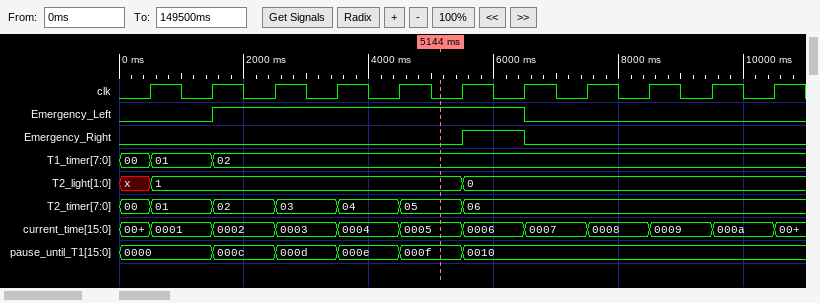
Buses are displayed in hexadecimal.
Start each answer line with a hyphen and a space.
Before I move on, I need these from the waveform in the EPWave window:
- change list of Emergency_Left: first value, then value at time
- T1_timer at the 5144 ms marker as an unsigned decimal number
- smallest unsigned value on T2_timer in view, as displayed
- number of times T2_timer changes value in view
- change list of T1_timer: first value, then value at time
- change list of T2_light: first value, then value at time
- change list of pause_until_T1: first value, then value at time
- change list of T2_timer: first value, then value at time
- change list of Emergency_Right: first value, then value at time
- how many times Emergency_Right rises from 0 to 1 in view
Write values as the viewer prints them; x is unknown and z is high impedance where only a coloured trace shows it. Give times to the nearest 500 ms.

- 0, 1 at 1500 ms, 0 at 6500 ms
- 2
- 00
- 6
- 00, 01 at 500 ms, 02 at 1500 ms
- x, 1 at 500 ms, 0 at 5500 ms
- 0000, 000c at 1500 ms, 000d at 2500 ms, 000e at 3500 ms, 000f at 4500 ms, 0010 at 5500 ms
- 00, 01 at 500 ms, 02 at 1500 ms, 03 at 2500 ms, 04 at 3500 ms, 05 at 4500 ms, 06 at 5500 ms
- 0, 1 at 5500 ms, 0 at 6500 ms
- 1
